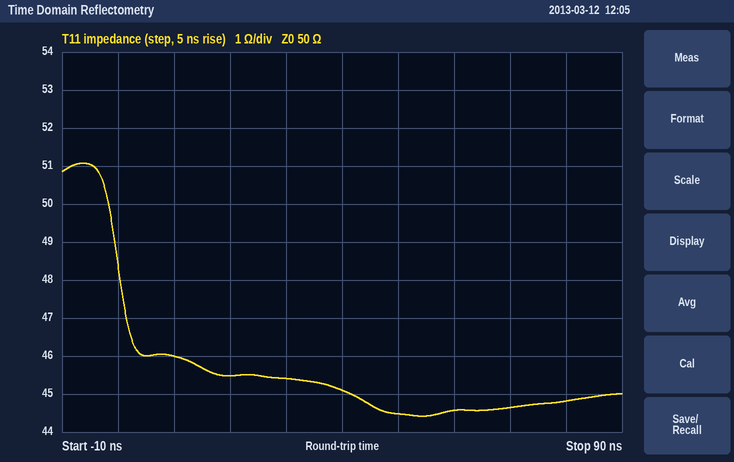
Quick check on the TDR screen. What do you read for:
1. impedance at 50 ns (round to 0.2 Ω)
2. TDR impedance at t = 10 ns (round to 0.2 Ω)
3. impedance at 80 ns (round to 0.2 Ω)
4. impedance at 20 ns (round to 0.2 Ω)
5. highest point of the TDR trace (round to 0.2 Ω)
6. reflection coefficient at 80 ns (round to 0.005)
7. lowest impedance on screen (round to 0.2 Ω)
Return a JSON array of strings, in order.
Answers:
["44.4 Ω", "46.0 Ω", "44.8 Ω", "45.4 Ω", "51.0 Ω", "-0.055", "44.4 Ω"]
